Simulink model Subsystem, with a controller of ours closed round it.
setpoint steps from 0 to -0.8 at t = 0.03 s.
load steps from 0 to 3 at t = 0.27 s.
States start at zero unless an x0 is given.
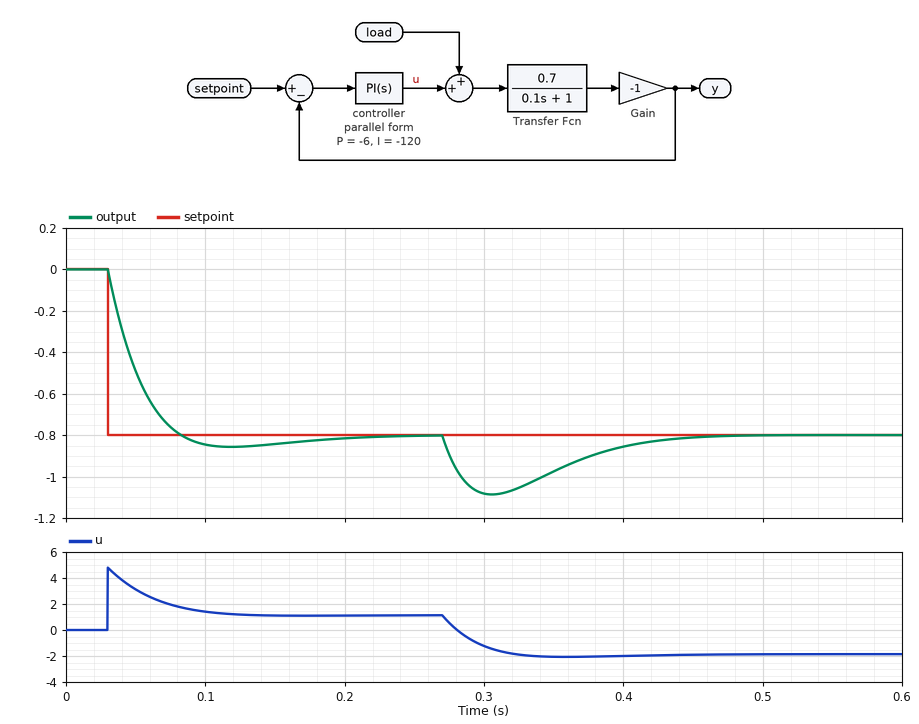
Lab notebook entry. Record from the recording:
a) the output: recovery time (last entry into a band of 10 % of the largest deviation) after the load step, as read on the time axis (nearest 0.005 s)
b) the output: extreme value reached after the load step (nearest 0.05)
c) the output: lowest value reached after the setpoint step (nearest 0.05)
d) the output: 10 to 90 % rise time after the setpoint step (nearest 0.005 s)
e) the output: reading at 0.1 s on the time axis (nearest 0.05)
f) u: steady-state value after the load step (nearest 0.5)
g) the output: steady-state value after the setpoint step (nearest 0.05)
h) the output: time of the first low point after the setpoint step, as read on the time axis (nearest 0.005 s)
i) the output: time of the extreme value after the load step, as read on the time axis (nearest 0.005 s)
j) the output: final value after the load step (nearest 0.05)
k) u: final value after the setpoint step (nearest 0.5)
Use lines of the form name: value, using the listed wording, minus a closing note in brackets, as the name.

the output: recovery time (last entry into a band of 10 % of the largest deviation) after the load step, as read on the time axis: 0.425 s
the output: extreme value reached after the load step: -1.10
the output: lowest value reached after the setpoint step: -0.85
the output: 10 to 90 % rise time after the setpoint step: 0.035 s
the output: reading at 0.1 s on the time axis: -0.85
u: steady-state value after the load step: -2.0
the output: steady-state value after the setpoint step: -0.80
the output: time of the first low point after the setpoint step, as read on the time axis: 0.120 s
the output: time of the extreme value after the load step, as read on the time axis: 0.305 s
the output: final value after the load step: -0.80
u: final value after the setpoint step: 1.0
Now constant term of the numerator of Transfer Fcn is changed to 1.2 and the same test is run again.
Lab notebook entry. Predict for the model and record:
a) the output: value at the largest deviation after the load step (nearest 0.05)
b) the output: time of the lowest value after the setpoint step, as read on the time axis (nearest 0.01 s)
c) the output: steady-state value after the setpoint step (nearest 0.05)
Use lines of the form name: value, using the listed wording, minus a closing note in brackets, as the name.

the output: value at the largest deviation after the load step: -1.15
the output: time of the lowest value after the setpoint step, as read on the time axis: 0.09 s
the output: steady-state value after the setpoint step: -0.80
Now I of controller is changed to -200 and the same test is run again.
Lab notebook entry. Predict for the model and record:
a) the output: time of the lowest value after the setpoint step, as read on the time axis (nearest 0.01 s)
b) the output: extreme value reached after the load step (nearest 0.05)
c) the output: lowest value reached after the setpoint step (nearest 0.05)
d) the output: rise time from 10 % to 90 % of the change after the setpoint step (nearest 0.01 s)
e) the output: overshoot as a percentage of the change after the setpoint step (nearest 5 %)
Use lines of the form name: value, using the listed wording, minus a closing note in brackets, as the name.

the output: time of the lowest value after the setpoint step, as read on the time axis: 0.10 s
the output: extreme value reached after the load step: -1.05
the output: lowest value reached after the setpoint step: -0.90
the output: rise time from 10 % to 90 % of the change after the setpoint step: 0.03 s
the output: overshoot as a percentage of the change after the setpoint step: 15 %
